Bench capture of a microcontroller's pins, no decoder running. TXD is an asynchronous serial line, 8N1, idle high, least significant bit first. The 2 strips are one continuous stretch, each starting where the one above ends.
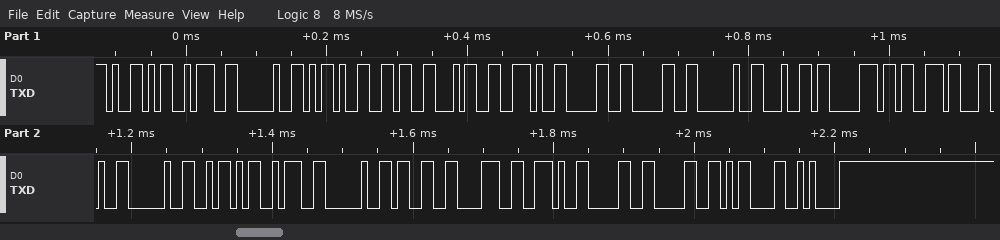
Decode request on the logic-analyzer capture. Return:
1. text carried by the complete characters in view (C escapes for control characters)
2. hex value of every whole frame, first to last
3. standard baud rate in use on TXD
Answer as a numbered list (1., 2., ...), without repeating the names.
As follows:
1. "Y: -64.00 dps, Z: 38.00\r\n"
2. 59 3A 20 2D 36 34 2E 30 30 20 64 70 73 2C 20 5A 3A 20 33 38 2E 30 30 0D 0A
3. 115200 baud
